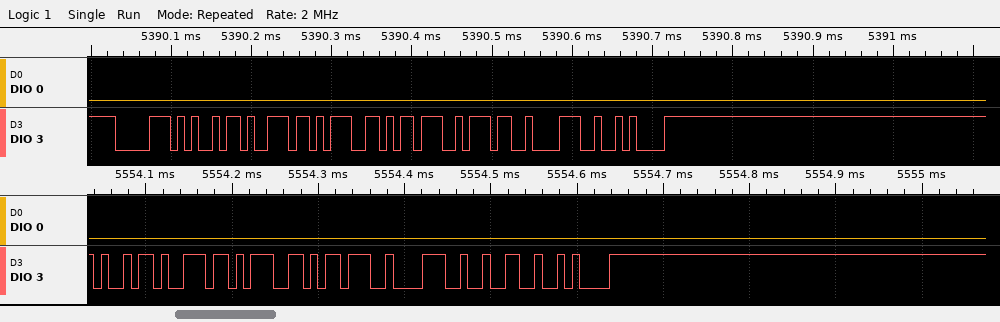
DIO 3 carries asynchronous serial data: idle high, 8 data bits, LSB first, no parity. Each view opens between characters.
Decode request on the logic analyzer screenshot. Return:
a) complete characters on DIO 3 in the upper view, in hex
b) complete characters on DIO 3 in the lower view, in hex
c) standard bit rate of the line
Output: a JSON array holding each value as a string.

["70, 69, 6E, 67, 3B, 37, 38, 0A", "69, 6E, 67, 3B, 38, 32, 0A", "115200 baud"]
